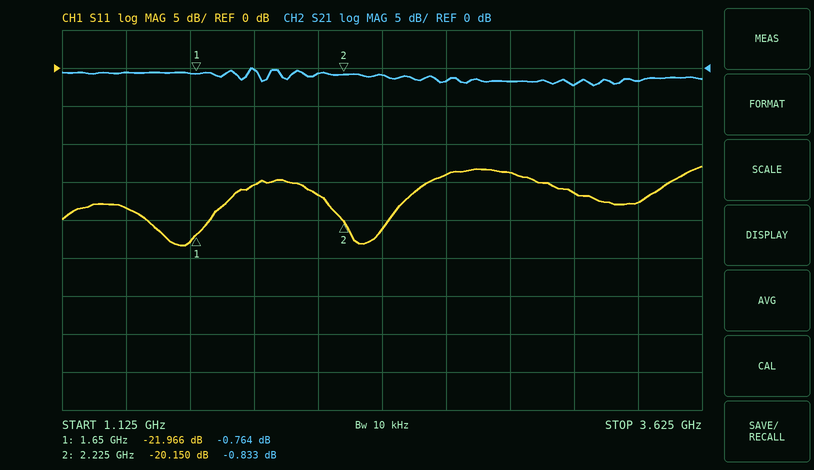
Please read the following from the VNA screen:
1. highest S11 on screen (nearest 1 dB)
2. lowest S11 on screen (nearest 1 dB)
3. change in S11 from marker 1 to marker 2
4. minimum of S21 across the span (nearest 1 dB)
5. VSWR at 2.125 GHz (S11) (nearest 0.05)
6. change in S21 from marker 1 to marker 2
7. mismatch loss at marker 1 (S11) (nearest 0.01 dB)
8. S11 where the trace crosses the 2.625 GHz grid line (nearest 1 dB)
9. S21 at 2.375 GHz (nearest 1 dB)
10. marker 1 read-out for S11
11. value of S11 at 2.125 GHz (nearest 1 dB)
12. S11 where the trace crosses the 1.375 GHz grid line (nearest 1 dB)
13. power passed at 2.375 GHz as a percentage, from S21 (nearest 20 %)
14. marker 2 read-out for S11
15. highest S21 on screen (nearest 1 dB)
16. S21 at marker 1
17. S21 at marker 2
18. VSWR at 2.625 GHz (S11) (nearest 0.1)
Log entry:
-13 dB
-23 dB
1.816 dB
-2 dB
1.35
-0.069 dB
0.03 dB
-14 dB
-1 dB
-21.966 dB
-17 dB
-18 dB
80 %
-20.150 dB
0 dB
-0.764 dB
-0.833 dB
1.5
